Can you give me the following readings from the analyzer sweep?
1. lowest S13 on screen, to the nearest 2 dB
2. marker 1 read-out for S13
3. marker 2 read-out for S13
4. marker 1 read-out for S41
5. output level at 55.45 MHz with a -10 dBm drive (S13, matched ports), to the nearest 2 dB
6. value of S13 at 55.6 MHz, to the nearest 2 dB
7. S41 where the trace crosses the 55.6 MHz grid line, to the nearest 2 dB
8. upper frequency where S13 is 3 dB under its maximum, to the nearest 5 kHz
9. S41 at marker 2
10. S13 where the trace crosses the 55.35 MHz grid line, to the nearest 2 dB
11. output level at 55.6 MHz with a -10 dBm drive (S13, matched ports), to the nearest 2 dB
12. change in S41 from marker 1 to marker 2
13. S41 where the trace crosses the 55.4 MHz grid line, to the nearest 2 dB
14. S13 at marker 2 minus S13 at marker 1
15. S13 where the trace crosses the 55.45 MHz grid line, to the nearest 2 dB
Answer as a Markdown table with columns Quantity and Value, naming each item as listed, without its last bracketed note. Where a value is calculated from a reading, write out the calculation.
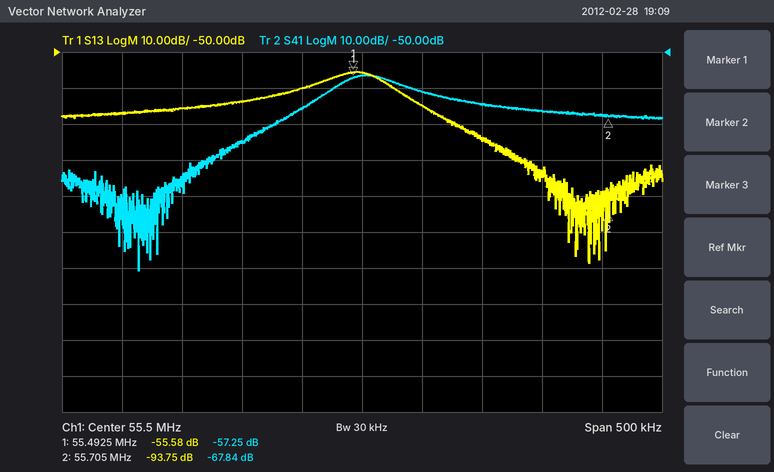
| Quantity | Value |
|---|---|
| lowest S13 on screen, to the nearest 2 dB | -108 dB |
| marker 1 read-out for S13 | -55.58 dB |
| marker 2 read-out for S13 | -93.75 dB |
| marker 1 read-out for S41 | -57.25 dB |
| output level at 55.45 MHz with a -10 dBm drive (S13, matched ports), to the nearest 2 dB | -10 dBm + (-60 dB) = -70 dBm |
| value of S13 at 55.6 MHz, to the nearest 2 dB | -74 dB |
| S41 where the trace crosses the 55.6 MHz grid line, to the nearest 2 dB | -64 dB |
| upper frequency where S13 is 3 dB under its maximum, to the nearest 5 kHz | 55.520 MHz |
| S41 at marker 2 | -67.84 dB |
| S13 where the trace crosses the 55.35 MHz grid line, to the nearest 2 dB | -66 dB |
| output level at 55.6 MHz with a -10 dBm drive (S13, matched ports), to the nearest 2 dB | -10 dBm + (-74 dB) = -84 dBm |
| change in S41 from marker 1 to marker 2 | -67.84 − (-57.25) = -10.59 dB |
| S41 where the trace crosses the 55.4 MHz grid line, to the nearest 2 dB | -74 dB |
| S13 at marker 2 minus S13 at marker 1 | -93.75 − (-55.58) = -38.17 dB |
| S13 where the trace crosses the 55.45 MHz grid line, to the nearest 2 dB | -60 dB |
